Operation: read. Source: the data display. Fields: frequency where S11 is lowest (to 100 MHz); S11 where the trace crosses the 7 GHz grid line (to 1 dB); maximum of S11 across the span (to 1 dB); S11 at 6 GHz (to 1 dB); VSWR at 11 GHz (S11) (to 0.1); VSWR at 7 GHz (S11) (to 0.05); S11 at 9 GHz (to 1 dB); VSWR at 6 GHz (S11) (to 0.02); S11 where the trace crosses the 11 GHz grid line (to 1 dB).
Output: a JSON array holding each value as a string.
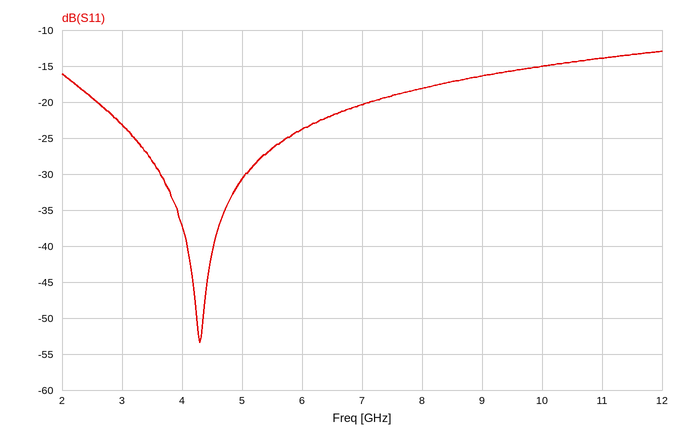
["4.3 GHz", "-20 dB", "-13 dB", "-24 dB", "1.5", "1.20", "-16 dB", "1.14", "-14 dB"]
